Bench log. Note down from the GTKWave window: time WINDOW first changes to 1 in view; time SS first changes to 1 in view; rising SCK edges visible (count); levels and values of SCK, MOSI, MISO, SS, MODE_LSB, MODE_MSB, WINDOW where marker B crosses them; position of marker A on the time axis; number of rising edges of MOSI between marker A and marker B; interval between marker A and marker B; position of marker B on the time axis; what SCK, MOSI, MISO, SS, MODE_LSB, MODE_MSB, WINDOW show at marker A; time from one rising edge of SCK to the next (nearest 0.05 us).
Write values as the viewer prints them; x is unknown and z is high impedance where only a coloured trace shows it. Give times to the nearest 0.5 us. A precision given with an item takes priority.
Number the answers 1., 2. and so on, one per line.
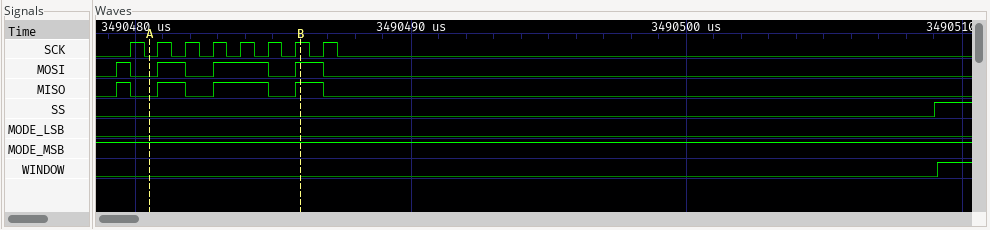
1. 3490509 us
2. 3490509 us
3. 8
4. SCK=1, MOSI=1, MISO=1, SS=0, MODE_LSB=0, MODE_MSB=1, WINDOW=0
5. 3490480.5 us
6. 3
7. 5.5 us
8. 3490486 us
9. SCK=0, MOSI=0, MISO=0, SS=0, MODE_LSB=0, MODE_MSB=1, WINDOW=0
10. 1 us
